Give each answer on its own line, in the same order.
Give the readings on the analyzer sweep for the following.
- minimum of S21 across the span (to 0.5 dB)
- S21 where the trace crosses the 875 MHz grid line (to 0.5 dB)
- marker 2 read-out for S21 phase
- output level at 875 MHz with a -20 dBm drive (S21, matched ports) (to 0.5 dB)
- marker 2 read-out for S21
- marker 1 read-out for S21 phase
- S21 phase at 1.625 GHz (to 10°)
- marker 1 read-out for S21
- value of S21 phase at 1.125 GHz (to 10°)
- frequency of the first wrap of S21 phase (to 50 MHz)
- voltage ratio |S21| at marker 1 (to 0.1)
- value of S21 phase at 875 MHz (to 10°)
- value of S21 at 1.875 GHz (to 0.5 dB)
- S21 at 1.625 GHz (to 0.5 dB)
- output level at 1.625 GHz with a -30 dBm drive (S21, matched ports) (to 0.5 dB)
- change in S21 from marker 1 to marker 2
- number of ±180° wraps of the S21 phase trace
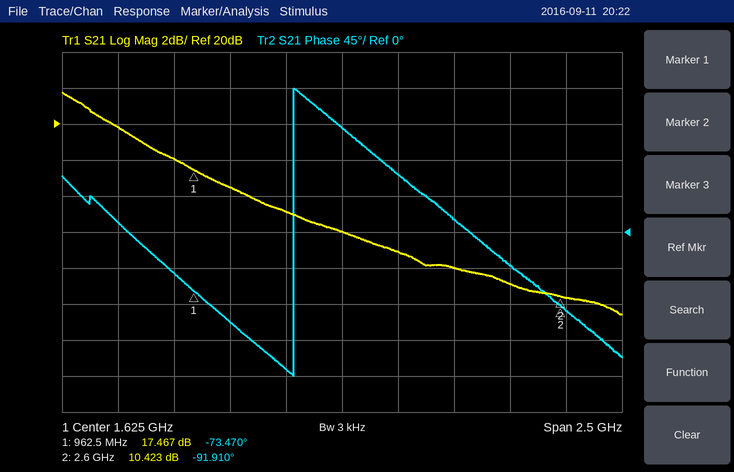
9.5 dB
18.0 dB
-91.910°
-2.0 dBm
10.423 dB
-73.470°
130°
17.467 dB
-110°
1.40 GHz
7.5
-50°
13.0 dB
14.0 dB
-16.0 dBm
-7.044 dB
1
